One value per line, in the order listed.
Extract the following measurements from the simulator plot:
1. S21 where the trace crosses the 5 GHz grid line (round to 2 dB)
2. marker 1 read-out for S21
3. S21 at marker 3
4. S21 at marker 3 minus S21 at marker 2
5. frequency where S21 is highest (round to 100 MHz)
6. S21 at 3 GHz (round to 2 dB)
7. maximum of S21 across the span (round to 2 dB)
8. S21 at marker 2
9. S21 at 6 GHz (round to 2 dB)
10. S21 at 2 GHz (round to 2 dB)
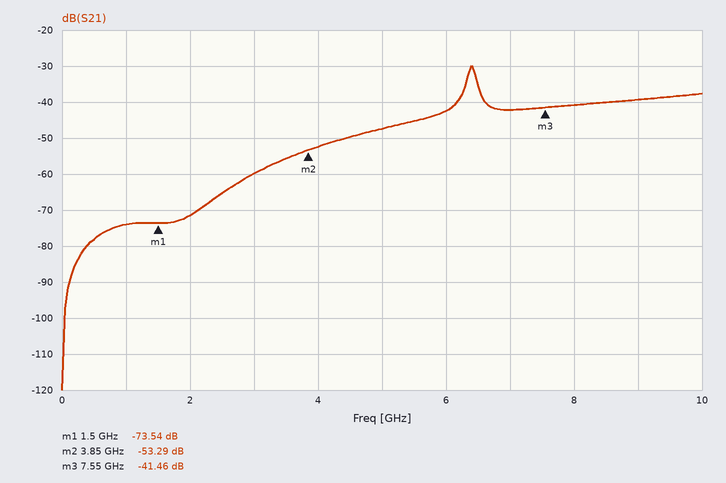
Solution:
-48 dB
-73.54 dB
-41.46 dB
11.83 dB
6.4 GHz
-60 dB
-30 dB
-53.29 dB
-42 dB
-72 dB
